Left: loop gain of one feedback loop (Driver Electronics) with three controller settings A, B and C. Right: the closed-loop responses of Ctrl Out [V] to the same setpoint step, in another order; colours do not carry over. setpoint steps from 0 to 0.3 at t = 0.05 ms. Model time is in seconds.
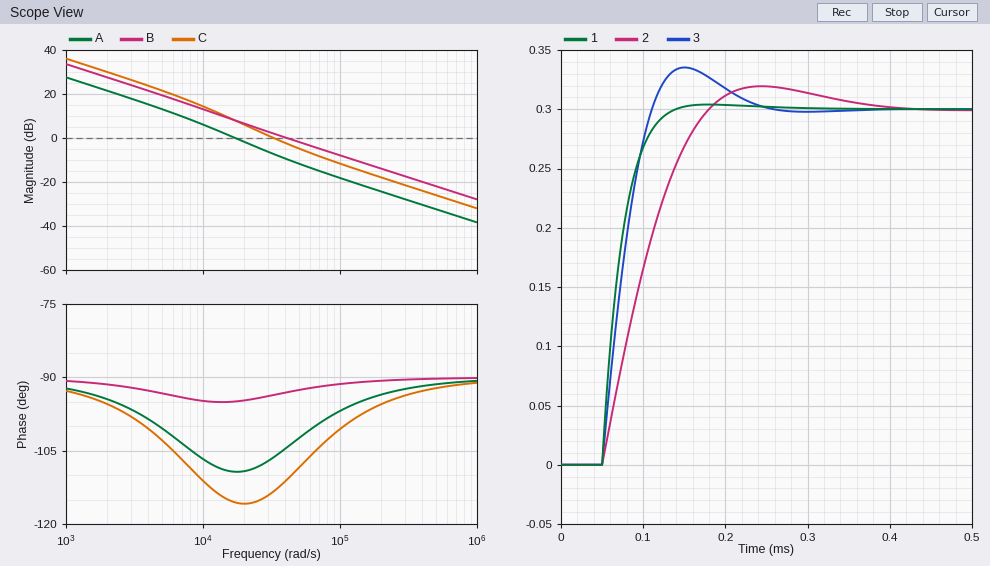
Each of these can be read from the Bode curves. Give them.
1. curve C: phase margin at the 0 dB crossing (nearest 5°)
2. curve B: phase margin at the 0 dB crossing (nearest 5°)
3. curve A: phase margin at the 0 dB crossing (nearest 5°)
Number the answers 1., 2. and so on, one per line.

1. 65°
2. 85°
3. 70°
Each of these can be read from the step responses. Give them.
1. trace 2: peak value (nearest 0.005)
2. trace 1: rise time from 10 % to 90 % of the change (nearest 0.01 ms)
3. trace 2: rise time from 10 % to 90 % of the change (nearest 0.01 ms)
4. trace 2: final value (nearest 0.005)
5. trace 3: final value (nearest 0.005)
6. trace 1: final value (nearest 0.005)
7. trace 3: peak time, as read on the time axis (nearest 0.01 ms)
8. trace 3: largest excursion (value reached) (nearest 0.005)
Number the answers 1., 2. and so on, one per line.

1. 0.320
2. 0.05 ms
3. 0.09 ms
4. 0.300
5. 0.300
6. 0.300
7. 0.15 ms
8. 0.335
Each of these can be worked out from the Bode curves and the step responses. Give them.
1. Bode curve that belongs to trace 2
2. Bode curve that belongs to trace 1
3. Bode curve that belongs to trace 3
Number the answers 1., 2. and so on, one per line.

1. A
2. B
3. C
